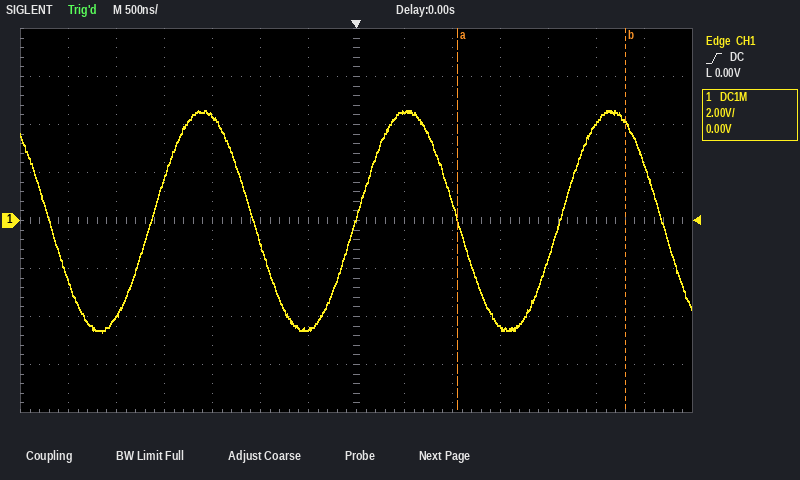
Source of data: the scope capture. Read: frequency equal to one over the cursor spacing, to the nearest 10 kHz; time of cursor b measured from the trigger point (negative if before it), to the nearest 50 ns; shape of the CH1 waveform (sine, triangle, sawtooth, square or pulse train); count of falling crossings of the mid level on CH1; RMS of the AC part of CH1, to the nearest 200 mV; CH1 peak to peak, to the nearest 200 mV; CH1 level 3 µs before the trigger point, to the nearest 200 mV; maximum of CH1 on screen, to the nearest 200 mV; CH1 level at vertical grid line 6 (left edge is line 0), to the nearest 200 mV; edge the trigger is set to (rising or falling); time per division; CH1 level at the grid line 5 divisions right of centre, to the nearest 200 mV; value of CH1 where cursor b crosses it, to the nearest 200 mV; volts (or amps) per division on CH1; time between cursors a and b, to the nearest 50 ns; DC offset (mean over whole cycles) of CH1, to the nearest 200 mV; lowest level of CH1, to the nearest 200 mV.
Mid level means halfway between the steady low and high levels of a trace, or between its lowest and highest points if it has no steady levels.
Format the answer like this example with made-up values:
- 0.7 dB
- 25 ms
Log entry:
- 570 kHz
- +2.80 µs
- sine
- 4
- 3.2 V
- 9.2 V
- -2.4 V
- 4.6 V
- -4.6 V
- rising
- 500 ns
- 4.0 V
- 4.0 V
- 2 V
- 1.75 µs
- 0.0 V
- -4.6 V
